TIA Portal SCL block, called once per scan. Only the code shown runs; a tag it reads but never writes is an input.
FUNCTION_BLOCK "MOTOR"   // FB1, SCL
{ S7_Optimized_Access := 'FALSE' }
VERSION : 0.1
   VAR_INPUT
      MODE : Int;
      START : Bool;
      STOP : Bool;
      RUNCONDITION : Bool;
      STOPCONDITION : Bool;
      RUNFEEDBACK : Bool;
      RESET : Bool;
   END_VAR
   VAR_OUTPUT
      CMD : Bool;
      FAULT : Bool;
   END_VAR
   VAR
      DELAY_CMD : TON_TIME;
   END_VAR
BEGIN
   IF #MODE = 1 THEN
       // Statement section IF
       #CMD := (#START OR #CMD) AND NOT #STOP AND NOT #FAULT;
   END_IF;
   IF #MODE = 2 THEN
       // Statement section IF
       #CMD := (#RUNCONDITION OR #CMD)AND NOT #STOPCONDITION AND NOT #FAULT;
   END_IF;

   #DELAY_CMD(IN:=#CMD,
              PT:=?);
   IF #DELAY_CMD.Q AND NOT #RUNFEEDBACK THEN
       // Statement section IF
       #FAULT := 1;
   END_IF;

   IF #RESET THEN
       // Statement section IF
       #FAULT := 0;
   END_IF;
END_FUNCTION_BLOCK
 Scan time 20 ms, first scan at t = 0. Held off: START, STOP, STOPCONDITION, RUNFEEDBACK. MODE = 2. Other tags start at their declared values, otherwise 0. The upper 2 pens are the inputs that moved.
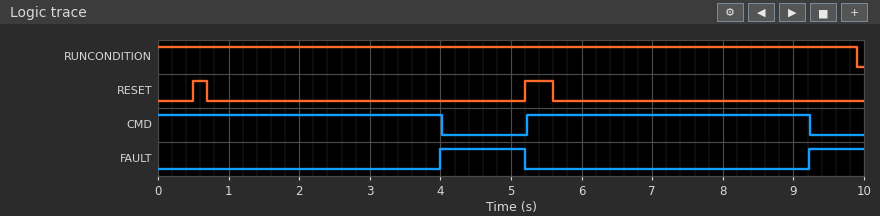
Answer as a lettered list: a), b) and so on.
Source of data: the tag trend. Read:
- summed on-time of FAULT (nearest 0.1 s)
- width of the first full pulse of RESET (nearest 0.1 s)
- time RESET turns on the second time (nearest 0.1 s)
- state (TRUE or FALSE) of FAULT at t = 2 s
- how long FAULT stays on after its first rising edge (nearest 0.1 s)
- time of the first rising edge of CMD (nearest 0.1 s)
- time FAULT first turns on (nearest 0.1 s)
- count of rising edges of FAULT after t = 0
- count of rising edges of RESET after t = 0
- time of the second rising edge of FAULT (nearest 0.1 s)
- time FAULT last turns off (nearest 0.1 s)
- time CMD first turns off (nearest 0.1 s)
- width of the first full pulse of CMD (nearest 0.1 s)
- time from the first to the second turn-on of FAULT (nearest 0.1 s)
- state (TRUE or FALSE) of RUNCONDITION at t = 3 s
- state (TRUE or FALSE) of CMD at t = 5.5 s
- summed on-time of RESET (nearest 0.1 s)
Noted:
a) 2.0 s
b) 0.2 s
c) 5.2 s
d) FALSE
e) 1.2 s
f) 5.2 s
g) 4.0 s
h) 2
i) 2
j) 9.2 s
k) 5.2 s
l) 4.0 s
m) 4.0 s
n) 5.2 s
o) TRUE
p) TRUE
q) 0.6 s
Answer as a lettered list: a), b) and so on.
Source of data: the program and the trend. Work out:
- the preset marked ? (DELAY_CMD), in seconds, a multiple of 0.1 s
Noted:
a) 4.0 s
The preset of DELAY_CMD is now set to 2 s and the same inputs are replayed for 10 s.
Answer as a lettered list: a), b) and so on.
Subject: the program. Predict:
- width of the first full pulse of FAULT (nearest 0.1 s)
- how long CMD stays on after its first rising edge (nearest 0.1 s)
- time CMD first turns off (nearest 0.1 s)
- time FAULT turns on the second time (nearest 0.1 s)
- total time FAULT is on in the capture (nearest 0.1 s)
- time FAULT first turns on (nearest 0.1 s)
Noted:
a) 3.2 s
b) 2.0 s
c) 2.0 s
d) 7.2 s
e) 6.0 s
f) 2.0 s
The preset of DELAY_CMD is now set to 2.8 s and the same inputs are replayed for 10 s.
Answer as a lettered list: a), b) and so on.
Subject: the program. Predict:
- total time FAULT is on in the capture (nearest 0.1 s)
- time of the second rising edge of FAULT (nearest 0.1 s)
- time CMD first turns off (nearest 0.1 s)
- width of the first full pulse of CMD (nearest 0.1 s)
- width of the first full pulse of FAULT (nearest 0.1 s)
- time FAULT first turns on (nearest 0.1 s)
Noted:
a) 4.4 s
b) 8.0 s
c) 2.8 s
d) 2.8 s
e) 2.4 s
f) 2.8 s
